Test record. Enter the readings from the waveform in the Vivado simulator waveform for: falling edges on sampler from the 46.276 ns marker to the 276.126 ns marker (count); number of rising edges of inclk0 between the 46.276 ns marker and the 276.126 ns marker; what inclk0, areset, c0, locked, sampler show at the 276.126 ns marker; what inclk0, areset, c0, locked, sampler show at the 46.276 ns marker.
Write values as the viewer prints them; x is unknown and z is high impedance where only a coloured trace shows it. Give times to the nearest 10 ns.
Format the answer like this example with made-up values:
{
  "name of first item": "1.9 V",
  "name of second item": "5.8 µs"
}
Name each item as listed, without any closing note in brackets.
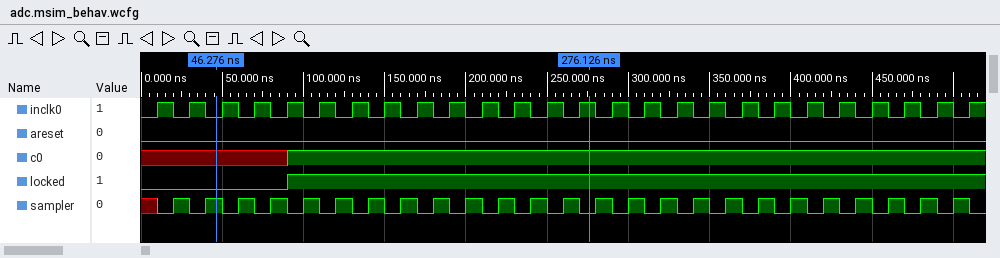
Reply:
{
  "falling edges on sampler from the 46.276 ns marker to the 276.126 ns marker": "12",
  "number of rising edges of inclk0 between the 46.276 ns marker and the 276.126 ns marker": "12",
  "what inclk0, areset, c0, locked, sampler show at the 276.126 ns marker": "inclk0=1, areset=0, c0=1, locked=1, sampler=0",
  "what inclk0, areset, c0, locked, sampler show at the 46.276 ns marker": "inclk0=0, areset=0, c0=x, locked=0, sampler=1"
}
